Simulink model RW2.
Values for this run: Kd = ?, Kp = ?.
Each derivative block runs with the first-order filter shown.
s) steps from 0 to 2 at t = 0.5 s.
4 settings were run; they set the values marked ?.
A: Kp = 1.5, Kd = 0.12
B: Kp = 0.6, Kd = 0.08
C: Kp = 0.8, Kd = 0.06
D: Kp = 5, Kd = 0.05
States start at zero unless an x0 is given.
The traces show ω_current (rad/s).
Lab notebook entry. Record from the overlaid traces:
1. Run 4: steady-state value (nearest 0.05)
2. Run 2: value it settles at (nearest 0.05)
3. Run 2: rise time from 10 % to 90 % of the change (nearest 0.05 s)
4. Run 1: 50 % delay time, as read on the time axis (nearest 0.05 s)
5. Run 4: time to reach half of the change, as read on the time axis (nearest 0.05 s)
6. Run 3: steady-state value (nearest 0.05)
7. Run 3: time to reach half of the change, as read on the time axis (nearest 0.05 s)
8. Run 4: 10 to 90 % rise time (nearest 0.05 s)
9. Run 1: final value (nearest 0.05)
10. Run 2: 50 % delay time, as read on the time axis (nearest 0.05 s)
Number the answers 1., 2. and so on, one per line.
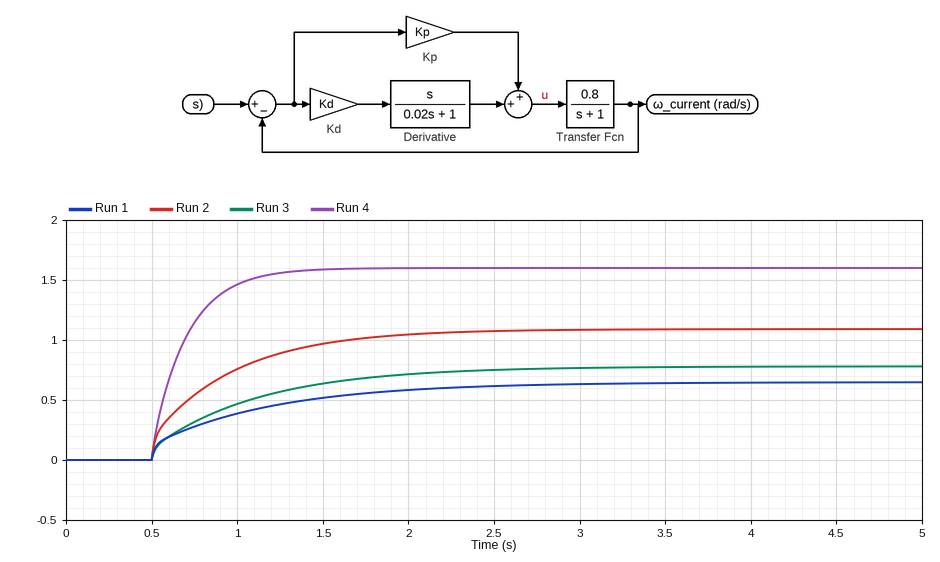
1. 1.60
2. 1.10
3. 1.05 s
4. 0.85 s
5. 0.65 s
6. 0.80
7. 0.85 s
8. 0.45 s
9. 0.65
10. 0.75 s
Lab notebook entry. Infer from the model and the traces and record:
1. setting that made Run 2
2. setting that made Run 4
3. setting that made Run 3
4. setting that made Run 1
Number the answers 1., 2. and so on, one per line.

1. A
2. D
3. C
4. B
